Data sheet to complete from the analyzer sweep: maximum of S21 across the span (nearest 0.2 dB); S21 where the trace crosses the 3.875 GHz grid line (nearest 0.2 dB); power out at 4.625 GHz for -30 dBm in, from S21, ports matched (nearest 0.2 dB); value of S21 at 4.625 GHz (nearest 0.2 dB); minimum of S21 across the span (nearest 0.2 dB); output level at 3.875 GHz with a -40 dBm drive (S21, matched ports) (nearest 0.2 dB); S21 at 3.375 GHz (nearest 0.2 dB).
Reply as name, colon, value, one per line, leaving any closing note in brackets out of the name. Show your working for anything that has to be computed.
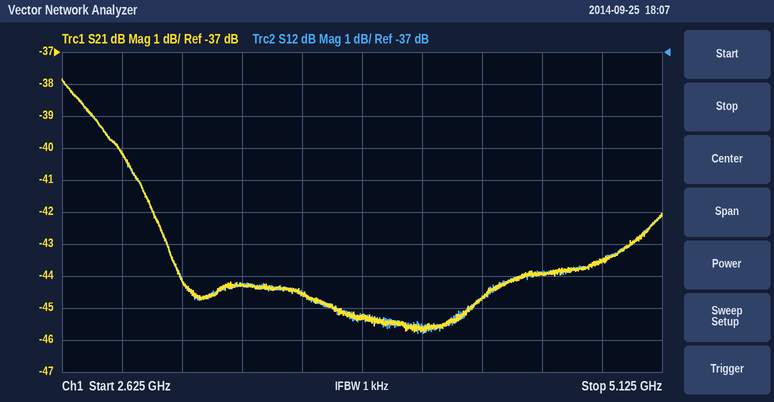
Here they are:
maximum of S21 across the span: -37.8 dB
S21 where the trace crosses the 3.875 GHz grid line: -45.2 dB
power out at 4.625 GHz for -30 dBm in, from S21, ports matched: -30 dBm + (-44.0 dB) = -74.0 dBm
value of S21 at 4.625 GHz: -44.0 dB
minimum of S21 across the span: -45.8 dB
output level at 3.875 GHz with a -40 dBm drive (S21, matched ports): -40 dBm + (-45.2 dB) = -85.2 dBm
S21 at 3.375 GHz: -44.2 dB
